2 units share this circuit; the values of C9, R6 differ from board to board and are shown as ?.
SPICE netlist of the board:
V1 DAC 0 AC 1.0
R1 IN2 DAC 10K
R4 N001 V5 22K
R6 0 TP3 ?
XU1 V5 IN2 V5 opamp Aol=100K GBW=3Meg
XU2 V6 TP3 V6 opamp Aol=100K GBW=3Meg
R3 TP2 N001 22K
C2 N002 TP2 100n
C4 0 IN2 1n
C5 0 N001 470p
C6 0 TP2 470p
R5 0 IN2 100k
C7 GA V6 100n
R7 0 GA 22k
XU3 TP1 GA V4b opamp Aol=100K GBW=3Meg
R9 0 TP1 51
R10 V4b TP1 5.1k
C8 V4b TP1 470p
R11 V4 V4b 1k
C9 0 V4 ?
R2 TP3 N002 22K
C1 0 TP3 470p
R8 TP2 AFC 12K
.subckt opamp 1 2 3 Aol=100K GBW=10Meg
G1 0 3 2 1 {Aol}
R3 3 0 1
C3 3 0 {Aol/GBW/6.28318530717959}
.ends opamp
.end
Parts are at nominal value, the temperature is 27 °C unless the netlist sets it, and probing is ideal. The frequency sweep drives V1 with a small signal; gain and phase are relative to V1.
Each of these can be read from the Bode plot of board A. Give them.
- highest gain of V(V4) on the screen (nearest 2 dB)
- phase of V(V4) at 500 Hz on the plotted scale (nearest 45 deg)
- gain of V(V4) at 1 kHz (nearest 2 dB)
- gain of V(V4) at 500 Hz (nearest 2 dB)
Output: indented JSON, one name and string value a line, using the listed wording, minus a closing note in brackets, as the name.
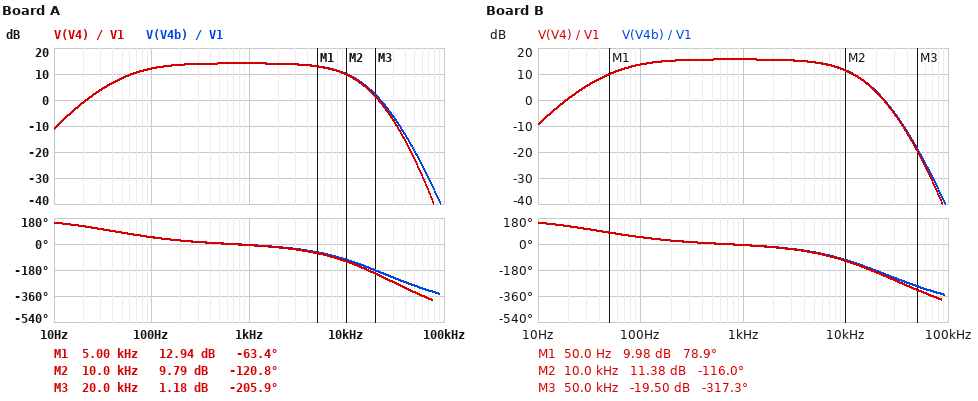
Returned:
{
  "highest gain of V(V4) on the screen": "14 dB",
  "phase of V(V4) at 500 Hz on the plotted scale": "0 deg",
  "gain of V(V4) at 1 kHz": "14 dB",
  "gain of V(V4) at 500 Hz": "14 dB"
}
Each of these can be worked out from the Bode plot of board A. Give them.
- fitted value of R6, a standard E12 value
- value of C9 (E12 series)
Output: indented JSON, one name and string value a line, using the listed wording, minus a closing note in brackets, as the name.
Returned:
{
  "fitted value of R6, a standard E12 value": "3.9 kΩ",
  "value of C9": "3.3 nF"
}
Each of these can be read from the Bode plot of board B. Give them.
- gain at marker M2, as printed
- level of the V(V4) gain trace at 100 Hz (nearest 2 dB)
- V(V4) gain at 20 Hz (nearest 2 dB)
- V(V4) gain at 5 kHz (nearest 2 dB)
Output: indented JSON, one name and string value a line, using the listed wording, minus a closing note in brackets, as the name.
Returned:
{
  "gain at marker M2, as printed": "11.38 dB",
  "level of the V(V4) gain trace at 100 Hz": "14 dB",
  "V(V4) gain at 20 Hz": "0 dB",
  "V(V4) gain at 5 kHz": "14 dB"
}
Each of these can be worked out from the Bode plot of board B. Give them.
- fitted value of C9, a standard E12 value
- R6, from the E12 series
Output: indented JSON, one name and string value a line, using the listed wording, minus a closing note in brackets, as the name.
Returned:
{
  "fitted value of C9, a standard E12 value": "1.5 nF",
  "R6, from the E12 series": "4.7 kΩ"
}
